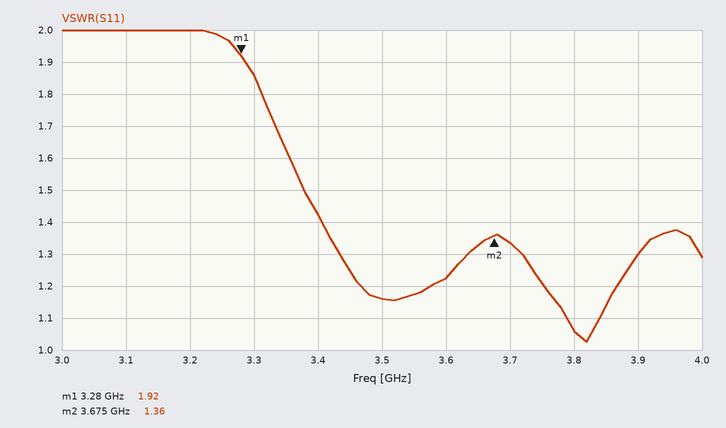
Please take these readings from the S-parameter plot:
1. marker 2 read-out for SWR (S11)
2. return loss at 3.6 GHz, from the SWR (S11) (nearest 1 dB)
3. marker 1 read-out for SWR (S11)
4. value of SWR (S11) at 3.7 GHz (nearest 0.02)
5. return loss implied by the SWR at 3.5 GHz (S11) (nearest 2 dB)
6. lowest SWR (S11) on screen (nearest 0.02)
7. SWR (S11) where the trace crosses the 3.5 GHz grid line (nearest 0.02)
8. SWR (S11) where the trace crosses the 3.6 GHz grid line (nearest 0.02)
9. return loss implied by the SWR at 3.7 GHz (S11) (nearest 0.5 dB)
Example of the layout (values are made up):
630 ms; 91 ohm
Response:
1.36; 20 dB; 1.92; 1.34; 22 dB; 1.02; 1.16; 1.22; 17.0 dB
